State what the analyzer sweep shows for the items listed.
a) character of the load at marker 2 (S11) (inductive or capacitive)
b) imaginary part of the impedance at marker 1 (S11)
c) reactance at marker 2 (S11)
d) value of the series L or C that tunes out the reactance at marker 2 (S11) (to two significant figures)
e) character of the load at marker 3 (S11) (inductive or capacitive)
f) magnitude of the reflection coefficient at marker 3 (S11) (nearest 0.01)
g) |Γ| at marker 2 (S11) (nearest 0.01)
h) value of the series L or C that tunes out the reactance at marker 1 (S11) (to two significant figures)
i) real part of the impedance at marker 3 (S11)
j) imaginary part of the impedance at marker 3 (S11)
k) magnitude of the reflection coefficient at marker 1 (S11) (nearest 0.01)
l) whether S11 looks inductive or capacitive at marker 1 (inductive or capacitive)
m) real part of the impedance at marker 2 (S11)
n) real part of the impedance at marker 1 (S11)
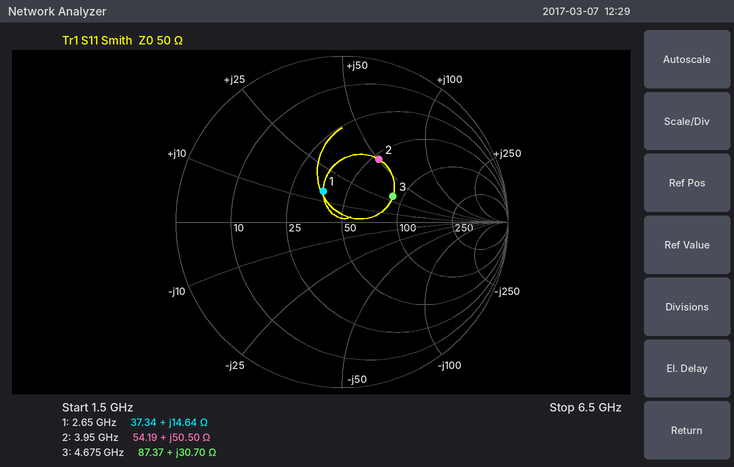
inductive
+14.64 Ω
+50.50 Ω
800 fF
inductive
0.34
0.44
4.1 pF
87.37 Ω
+30.70 Ω
0.22
inductive
54.19 Ω
37.34 Ω
